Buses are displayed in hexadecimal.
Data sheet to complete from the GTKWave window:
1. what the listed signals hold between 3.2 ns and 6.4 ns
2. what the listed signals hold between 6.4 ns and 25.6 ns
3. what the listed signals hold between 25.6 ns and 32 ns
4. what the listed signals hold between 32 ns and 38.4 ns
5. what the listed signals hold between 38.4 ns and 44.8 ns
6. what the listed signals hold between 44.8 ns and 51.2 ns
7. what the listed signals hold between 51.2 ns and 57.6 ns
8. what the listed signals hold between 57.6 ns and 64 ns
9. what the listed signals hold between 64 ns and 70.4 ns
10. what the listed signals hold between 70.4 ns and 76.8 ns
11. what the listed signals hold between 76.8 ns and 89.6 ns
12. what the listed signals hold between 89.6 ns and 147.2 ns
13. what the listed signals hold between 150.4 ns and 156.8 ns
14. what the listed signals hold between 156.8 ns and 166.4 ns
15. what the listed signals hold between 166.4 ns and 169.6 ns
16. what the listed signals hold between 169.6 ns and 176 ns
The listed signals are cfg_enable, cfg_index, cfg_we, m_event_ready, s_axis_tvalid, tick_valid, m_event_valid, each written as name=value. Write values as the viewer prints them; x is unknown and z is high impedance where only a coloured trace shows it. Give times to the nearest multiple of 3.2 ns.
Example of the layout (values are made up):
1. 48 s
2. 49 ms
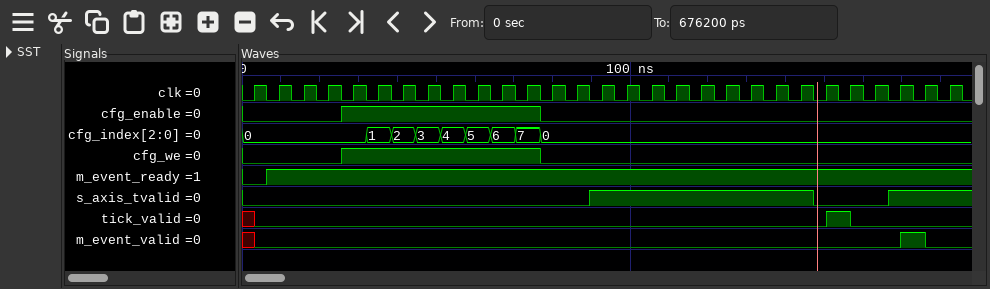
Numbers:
1. cfg_enable=0, cfg_index=0, cfg_we=0, m_event_ready=0, s_axis_tvalid=0, tick_valid=0, m_event_valid=0
2. cfg_enable=0, cfg_index=0, cfg_we=0, m_event_ready=1, s_axis_tvalid=0, tick_valid=0, m_event_valid=0
3. cfg_enable=1, cfg_index=0, cfg_we=1, m_event_ready=1, s_axis_tvalid=0, tick_valid=0, m_event_valid=0
4. cfg_enable=1, cfg_index=1, cfg_we=1, m_event_ready=1, s_axis_tvalid=0, tick_valid=0, m_event_valid=0
5. cfg_enable=1, cfg_index=2, cfg_we=1, m_event_ready=1, s_axis_tvalid=0, tick_valid=0, m_event_valid=0
6. cfg_enable=1, cfg_index=3, cfg_we=1, m_event_ready=1, s_axis_tvalid=0, tick_valid=0, m_event_valid=0
7. cfg_enable=1, cfg_index=4, cfg_we=1, m_event_ready=1, s_axis_tvalid=0, tick_valid=0, m_event_valid=0
8. cfg_enable=1, cfg_index=5, cfg_we=1, m_event_ready=1, s_axis_tvalid=0, tick_valid=0, m_event_valid=0
9. cfg_enable=1, cfg_index=6, cfg_we=1, m_event_ready=1, s_axis_tvalid=0, tick_valid=0, m_event_valid=0
10. cfg_enable=1, cfg_index=7, cfg_we=1, m_event_ready=1, s_axis_tvalid=0, tick_valid=0, m_event_valid=0
11. cfg_enable=0, cfg_index=0, cfg_we=0, m_event_ready=1, s_axis_tvalid=0, tick_valid=0, m_event_valid=0
12. cfg_enable=0, cfg_index=0, cfg_we=0, m_event_ready=1, s_axis_tvalid=1, tick_valid=0, m_event_valid=0
13. cfg_enable=0, cfg_index=0, cfg_we=0, m_event_ready=1, s_axis_tvalid=0, tick_valid=1, m_event_valid=0
14. cfg_enable=0, cfg_index=0, cfg_we=0, m_event_ready=1, s_axis_tvalid=0, tick_valid=0, m_event_valid=0
15. cfg_enable=0, cfg_index=0, cfg_we=0, m_event_ready=1, s_axis_tvalid=1, tick_valid=0, m_event_valid=0
16. cfg_enable=0, cfg_index=0, cfg_we=0, m_event_ready=1, s_axis_tvalid=1, tick_valid=0, m_event_valid=1
